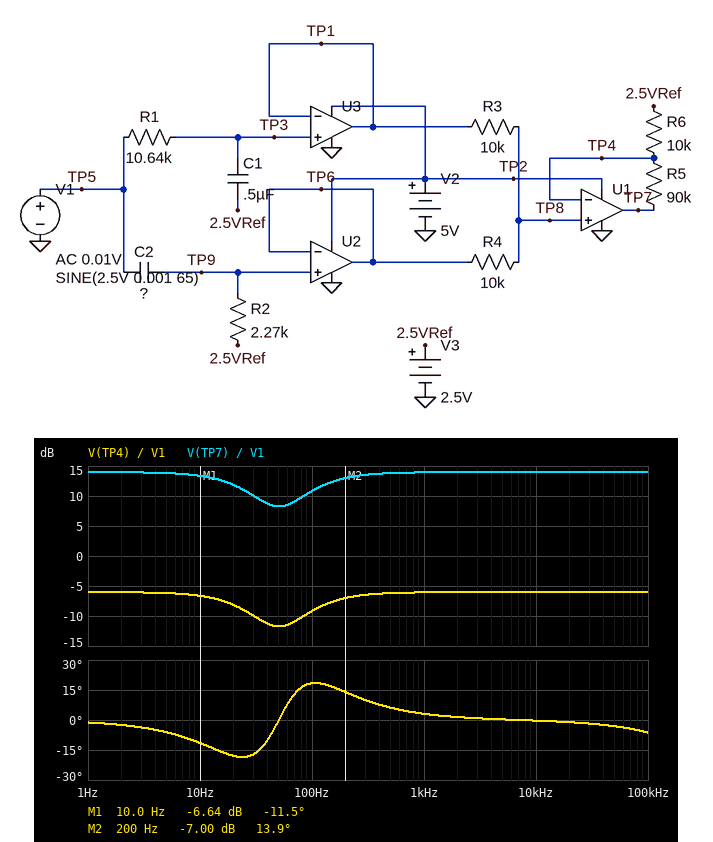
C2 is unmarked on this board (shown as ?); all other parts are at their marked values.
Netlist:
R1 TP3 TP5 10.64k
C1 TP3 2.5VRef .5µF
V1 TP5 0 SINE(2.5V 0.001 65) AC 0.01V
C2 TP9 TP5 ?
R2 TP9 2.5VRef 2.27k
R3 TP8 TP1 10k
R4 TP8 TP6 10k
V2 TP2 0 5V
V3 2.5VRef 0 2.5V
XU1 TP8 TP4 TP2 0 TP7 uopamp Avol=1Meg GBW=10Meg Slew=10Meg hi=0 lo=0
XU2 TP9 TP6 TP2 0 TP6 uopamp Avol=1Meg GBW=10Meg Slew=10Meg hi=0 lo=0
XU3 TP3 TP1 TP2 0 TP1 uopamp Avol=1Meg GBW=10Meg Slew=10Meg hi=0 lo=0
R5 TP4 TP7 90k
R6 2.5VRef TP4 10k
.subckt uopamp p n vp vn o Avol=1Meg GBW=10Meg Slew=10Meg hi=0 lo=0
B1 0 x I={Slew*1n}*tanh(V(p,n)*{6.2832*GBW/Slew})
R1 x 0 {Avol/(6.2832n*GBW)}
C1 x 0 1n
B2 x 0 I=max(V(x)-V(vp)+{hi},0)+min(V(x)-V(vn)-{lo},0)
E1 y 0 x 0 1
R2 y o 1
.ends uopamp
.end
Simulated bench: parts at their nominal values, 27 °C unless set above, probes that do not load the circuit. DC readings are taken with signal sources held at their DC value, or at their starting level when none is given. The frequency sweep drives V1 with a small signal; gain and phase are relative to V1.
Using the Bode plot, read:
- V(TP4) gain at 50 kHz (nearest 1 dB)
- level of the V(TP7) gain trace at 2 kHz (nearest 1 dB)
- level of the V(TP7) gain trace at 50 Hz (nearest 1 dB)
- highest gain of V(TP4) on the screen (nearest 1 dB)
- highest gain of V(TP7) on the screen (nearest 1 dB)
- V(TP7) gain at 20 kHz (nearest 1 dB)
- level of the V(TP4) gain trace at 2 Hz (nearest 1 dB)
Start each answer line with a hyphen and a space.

- -6 dB
- 14 dB
- 8 dB
- -6 dB
- 14 dB
- 14 dB
- -6 dB
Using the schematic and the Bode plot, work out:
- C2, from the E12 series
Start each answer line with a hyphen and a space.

- 820 nF
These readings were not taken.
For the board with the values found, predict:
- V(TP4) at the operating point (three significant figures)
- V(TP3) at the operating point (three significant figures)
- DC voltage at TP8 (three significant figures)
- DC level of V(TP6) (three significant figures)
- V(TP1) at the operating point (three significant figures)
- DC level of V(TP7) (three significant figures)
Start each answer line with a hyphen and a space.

- 2.50 V
- 2.50 V
- 2.50 V
- 2.50 V
- 2.50 V
- 2.50 V
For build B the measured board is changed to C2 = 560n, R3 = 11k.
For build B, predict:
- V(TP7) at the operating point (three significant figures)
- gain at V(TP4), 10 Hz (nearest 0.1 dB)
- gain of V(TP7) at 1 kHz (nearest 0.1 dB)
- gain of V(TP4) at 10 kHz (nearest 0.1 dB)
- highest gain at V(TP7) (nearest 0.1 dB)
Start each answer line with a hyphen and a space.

- 2.50 V
- -7.1 dB
- 14.3 dB
- -5.6 dB
- 14.4 dB
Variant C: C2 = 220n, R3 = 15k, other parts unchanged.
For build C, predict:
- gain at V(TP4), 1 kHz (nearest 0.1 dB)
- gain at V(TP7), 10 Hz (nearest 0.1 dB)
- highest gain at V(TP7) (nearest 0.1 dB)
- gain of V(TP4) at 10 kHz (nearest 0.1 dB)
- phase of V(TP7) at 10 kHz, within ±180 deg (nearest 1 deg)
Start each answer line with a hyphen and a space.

- -4.9 dB
- 11.5 dB
- 15.6 dB
- -4.4 dB
- 1 deg
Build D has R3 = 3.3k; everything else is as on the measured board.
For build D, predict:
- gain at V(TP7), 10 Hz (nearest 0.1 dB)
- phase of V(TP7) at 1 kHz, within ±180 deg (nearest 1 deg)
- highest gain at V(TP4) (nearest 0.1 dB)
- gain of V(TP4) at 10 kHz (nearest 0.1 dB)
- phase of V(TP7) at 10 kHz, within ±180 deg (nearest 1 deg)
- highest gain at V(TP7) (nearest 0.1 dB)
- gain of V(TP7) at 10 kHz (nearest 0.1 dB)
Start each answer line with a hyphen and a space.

- 17.0 dB
- 0 deg
- -2.5 dB
- -12.1 dB
- -1 deg
- 17.5 dB
- 7.9 dB
